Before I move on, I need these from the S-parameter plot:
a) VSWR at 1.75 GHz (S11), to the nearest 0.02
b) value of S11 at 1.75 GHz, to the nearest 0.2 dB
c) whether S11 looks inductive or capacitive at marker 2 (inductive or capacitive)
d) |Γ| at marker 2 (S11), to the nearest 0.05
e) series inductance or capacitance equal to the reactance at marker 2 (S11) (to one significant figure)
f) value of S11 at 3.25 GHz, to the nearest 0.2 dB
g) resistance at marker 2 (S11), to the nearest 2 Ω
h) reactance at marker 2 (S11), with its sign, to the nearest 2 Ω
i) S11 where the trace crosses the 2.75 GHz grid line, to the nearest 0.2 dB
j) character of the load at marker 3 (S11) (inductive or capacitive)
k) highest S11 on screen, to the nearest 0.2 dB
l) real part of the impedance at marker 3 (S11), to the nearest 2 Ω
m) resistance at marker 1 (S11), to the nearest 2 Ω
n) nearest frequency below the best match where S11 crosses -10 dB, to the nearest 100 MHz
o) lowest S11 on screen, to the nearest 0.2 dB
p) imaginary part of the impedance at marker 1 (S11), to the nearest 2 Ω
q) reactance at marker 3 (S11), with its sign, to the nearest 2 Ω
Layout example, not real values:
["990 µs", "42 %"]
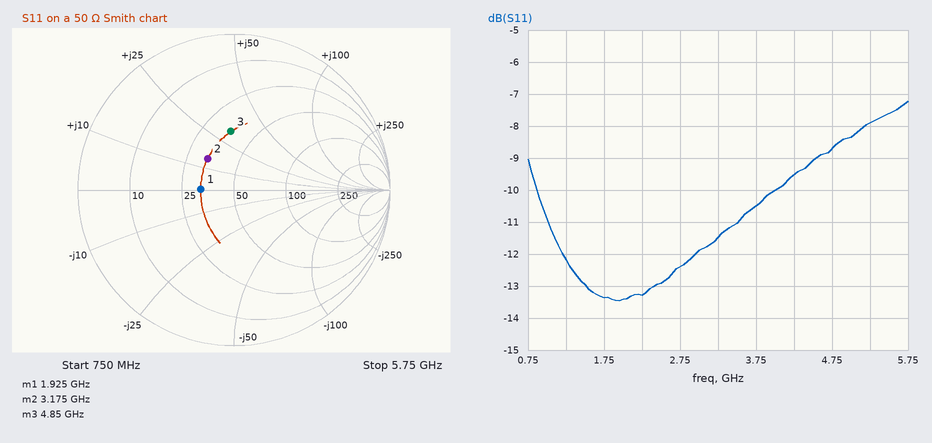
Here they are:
["1.54", "-13.4 dB", "inductive", "0.25", "700 pH", "-11.4 dB", "34 Ω", "+14 Ω", "-12.4 dB", "inductive", "-7.2 dB", "36 Ω", "32 Ω", "900 MHz", "-13.4 dB", "0 Ω", "+32 Ω"]
